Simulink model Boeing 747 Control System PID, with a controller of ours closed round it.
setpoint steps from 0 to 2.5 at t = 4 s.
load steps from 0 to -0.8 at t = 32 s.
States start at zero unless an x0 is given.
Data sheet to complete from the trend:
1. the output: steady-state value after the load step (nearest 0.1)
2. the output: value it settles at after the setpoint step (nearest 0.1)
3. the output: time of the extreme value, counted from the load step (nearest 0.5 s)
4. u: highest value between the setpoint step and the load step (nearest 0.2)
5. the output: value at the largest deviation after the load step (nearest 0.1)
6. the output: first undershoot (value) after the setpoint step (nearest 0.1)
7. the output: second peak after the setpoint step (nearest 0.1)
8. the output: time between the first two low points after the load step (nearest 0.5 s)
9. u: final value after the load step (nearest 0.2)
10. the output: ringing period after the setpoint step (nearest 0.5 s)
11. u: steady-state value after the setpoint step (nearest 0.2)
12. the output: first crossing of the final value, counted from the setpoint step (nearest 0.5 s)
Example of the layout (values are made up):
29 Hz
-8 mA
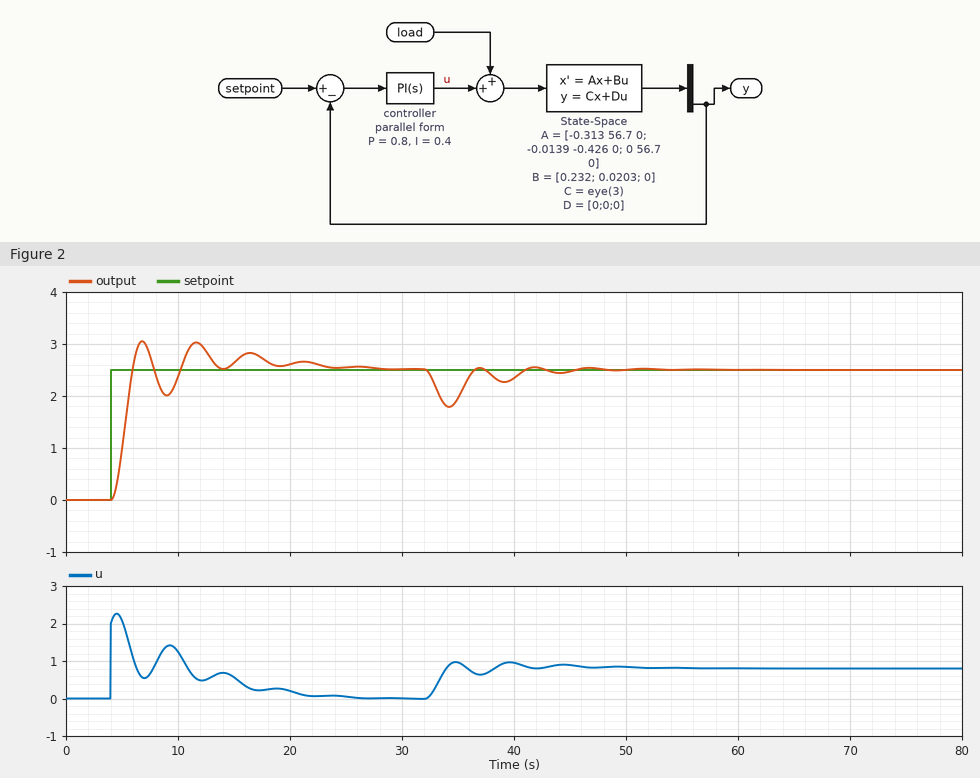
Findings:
2.5
2.5
2.0 s
2.2
1.8
2.0
3.0
5.0 s
0.8
5.0 s
0.0
2.0 s
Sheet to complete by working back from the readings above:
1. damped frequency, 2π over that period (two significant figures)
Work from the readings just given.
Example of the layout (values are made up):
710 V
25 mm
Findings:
1.3 rad/s
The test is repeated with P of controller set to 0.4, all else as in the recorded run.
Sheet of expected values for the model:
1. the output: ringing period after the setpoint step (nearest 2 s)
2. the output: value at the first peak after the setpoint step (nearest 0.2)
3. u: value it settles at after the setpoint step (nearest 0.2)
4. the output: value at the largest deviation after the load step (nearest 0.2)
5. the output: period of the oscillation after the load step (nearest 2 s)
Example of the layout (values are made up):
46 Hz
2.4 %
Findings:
6 s
3.2
0.0
1.6
6 s
